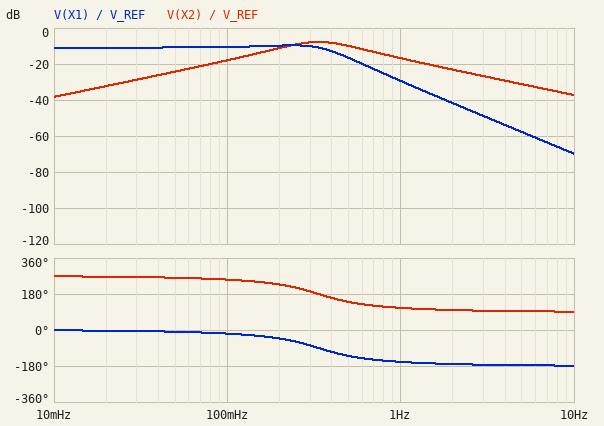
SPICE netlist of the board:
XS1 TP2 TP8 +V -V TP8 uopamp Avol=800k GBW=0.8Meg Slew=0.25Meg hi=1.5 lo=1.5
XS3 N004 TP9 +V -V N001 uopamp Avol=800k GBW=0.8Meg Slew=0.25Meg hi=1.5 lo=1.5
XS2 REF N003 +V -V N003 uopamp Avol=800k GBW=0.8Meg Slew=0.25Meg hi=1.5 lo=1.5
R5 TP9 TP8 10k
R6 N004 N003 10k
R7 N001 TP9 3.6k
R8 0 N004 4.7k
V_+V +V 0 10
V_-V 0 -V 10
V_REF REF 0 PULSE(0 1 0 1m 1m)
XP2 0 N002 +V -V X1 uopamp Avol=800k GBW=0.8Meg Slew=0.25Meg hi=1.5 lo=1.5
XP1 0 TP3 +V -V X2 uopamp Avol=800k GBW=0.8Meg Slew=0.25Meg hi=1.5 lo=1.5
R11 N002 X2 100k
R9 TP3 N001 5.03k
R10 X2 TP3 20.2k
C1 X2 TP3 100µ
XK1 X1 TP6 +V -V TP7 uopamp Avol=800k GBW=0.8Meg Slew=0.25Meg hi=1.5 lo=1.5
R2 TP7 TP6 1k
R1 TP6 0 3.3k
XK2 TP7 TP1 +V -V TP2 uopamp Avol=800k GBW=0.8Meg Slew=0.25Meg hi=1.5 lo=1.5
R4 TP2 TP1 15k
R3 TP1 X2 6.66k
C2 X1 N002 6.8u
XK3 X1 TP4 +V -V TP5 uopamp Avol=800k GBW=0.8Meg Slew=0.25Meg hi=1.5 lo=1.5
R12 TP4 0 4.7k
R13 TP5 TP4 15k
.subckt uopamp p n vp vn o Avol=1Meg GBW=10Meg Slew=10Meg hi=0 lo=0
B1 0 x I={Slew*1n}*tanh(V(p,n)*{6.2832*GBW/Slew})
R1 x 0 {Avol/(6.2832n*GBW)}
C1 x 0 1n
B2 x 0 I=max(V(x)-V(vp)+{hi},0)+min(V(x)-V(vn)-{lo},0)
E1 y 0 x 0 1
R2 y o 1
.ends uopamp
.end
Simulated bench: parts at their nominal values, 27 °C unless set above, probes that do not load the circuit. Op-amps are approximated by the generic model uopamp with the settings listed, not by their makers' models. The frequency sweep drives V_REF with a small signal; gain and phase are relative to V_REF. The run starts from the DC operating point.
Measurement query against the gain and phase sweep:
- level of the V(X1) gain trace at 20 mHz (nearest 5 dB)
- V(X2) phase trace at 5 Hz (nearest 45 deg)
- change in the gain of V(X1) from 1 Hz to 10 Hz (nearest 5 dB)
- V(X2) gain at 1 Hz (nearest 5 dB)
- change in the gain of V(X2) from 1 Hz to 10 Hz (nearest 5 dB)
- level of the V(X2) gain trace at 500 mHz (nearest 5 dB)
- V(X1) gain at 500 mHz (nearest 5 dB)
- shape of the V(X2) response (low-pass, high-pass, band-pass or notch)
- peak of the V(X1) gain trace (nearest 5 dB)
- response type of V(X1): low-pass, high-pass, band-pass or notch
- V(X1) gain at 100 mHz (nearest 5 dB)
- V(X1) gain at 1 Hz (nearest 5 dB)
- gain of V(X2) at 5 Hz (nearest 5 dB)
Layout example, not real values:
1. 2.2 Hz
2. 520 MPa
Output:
1. -10 dB
2. 90 deg
3. -40 dB
4. -15 dB
5. -20 dB
6. -10 dB
7. -15 dB
8. band-pass
9. -10 dB
10. low-pass
11. -10 dB
12. -30 dB
13. -30 dB
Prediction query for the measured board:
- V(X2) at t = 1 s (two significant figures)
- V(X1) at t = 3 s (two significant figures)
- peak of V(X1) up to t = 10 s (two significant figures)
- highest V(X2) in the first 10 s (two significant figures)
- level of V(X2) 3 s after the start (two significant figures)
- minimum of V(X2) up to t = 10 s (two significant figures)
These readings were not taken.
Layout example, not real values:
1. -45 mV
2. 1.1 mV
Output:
1. -160 mV
2. 280 mV
3. 330 mV
4. 37 mV
5. 14 mV
6. -220 mV
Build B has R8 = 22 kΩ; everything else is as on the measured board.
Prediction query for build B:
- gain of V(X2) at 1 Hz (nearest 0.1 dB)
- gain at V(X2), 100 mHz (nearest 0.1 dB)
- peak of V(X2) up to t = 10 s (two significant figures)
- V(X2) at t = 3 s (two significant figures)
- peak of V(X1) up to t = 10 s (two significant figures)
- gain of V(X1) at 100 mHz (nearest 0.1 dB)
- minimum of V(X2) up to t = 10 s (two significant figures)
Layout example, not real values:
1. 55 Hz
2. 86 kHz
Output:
1. -10.1 dB
2. -11.3 dB
3. 79 mV
4. 31 mV
5. 710 mV
6. -3.9 dB
7. -480 mV
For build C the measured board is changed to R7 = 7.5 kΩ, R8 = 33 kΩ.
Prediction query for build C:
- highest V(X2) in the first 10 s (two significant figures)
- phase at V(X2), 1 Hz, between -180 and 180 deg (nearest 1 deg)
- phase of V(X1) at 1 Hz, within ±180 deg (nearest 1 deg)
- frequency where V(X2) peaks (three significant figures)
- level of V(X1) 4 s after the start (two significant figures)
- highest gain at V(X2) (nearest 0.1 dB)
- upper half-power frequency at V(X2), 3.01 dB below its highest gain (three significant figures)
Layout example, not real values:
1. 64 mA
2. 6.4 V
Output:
1. 33 mV
2. 129 deg
3. -141 deg
4. 485 mHz
5. 420 mV
6. -3.2 dB
7. 881 mHz
